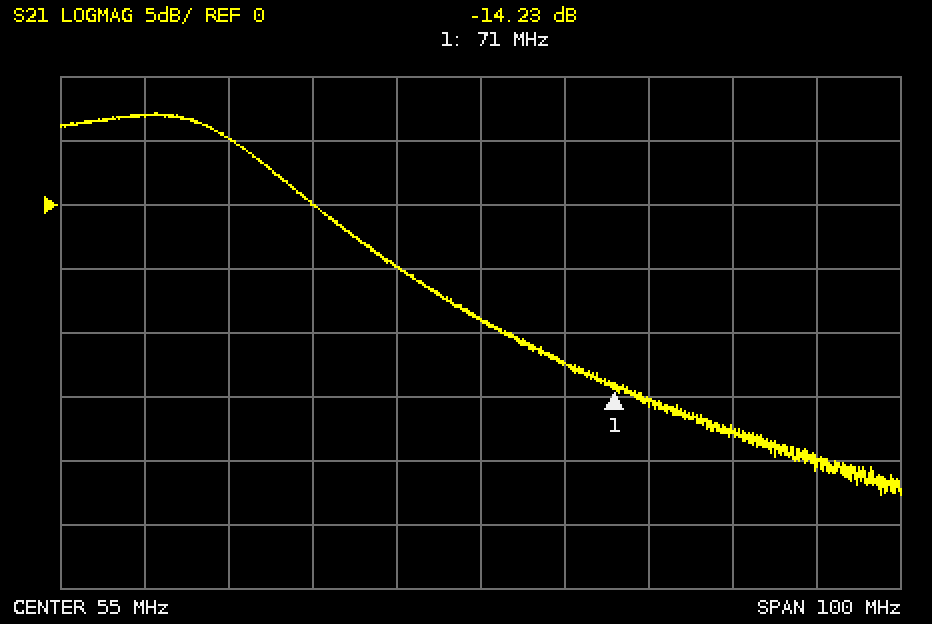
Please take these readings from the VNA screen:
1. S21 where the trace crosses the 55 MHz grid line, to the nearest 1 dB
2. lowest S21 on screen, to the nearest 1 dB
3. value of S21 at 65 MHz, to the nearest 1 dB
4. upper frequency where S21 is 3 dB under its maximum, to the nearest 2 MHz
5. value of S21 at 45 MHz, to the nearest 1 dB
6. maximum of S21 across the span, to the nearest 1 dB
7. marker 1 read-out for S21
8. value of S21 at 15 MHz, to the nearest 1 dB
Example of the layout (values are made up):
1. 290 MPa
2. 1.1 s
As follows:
1. -9 dB
2. -23 dB
3. -12 dB
4. 28 MHz
5. -5 dB
6. 7 dB
7. -14.23 dB
8. 7 dB
